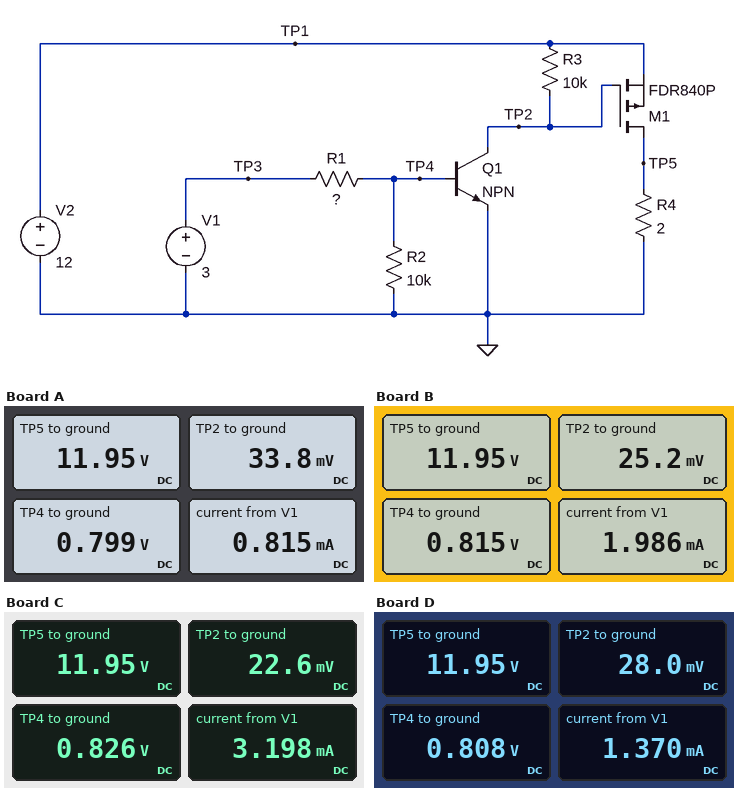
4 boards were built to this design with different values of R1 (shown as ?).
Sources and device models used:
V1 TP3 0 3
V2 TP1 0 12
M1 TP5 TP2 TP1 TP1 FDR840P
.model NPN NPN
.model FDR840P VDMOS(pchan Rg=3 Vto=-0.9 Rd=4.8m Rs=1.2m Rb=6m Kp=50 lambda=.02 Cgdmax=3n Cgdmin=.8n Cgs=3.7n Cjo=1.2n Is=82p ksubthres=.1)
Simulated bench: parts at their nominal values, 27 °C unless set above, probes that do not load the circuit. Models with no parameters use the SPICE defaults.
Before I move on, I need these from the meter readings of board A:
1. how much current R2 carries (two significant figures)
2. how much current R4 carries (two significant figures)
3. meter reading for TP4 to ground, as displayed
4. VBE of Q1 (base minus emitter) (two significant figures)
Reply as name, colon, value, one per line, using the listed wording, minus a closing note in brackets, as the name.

how much current R2 carries: 80 µA
how much current R4 carries: 6.0 A
meter reading for TP4 to ground, as displayed: 0.799 V
VBE of Q1 (base minus emitter): 800 mV
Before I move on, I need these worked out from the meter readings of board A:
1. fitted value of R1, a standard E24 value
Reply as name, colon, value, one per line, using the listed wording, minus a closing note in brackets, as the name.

fitted value of R1, a standard E24 value: 2.7 kΩ
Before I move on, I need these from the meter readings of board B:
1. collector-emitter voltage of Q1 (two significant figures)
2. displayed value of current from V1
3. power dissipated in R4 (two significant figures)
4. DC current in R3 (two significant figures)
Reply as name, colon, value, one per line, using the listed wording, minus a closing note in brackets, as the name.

collector-emitter voltage of Q1: 25 mV
displayed value of current from V1: 1.986 mA
power dissipated in R4: 71 W
DC current in R3: 1.2 mA
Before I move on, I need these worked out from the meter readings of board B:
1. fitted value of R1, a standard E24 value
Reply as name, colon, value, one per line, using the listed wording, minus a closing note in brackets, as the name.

fitted value of R1, a standard E24 value: 1.1 kΩ
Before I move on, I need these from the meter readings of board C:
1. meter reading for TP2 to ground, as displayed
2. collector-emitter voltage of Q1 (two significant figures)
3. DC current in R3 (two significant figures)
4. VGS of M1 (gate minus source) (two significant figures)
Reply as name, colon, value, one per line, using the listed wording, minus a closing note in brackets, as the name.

meter reading for TP2 to ground, as displayed: 22.6 mV
collector-emitter voltage of Q1: 23 mV
DC current in R3: 1.2 mA
VGS of M1 (gate minus source): -12 V
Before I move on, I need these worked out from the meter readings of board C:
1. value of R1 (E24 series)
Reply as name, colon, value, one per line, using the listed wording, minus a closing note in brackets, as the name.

value of R1: 680 Ω
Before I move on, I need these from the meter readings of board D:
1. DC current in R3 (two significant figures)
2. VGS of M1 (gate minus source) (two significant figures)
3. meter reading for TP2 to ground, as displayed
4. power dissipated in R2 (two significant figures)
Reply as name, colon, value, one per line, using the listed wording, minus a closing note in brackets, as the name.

DC current in R3: 1.2 mA
VGS of M1 (gate minus source): -12 V
meter reading for TP2 to ground, as displayed: 28.0 mV
power dissipated in R2: 65 µW
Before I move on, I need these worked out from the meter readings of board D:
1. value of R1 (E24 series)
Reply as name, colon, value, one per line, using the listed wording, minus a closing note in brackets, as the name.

value of R1: 1.6 kΩ
